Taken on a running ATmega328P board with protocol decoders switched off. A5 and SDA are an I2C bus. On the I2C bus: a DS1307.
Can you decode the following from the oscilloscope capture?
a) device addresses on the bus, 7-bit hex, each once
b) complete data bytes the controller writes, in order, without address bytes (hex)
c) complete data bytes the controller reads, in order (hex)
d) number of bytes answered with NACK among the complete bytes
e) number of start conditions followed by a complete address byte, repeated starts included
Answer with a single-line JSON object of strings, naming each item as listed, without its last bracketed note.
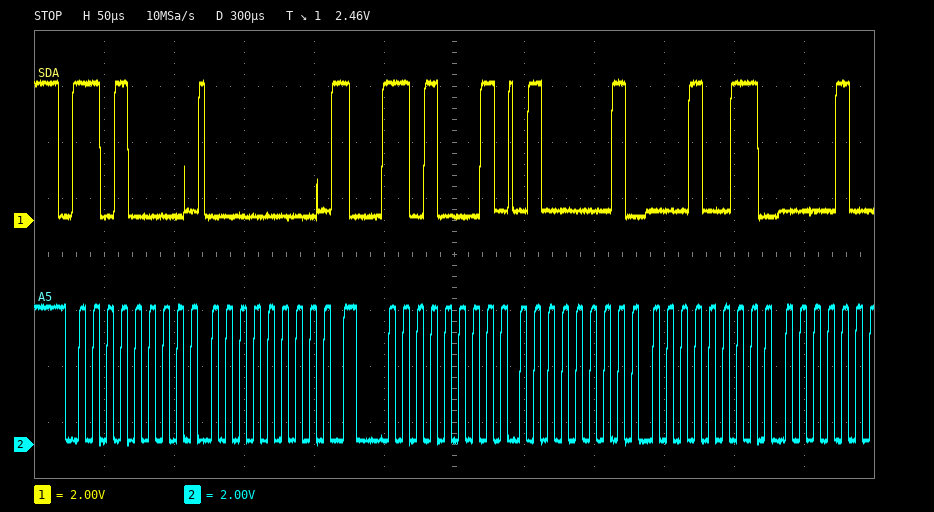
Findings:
{"device addresses on the bus, 7-bit hex, each once": "0x68", "complete data bytes the controller writes, in order, without address bytes": "00", "complete data bytes the controller reads, in order": "41 13", "number of bytes answered with NACK among the complete bytes": "0", "number of start conditions followed by a complete address byte, repeated starts included": "2"}
